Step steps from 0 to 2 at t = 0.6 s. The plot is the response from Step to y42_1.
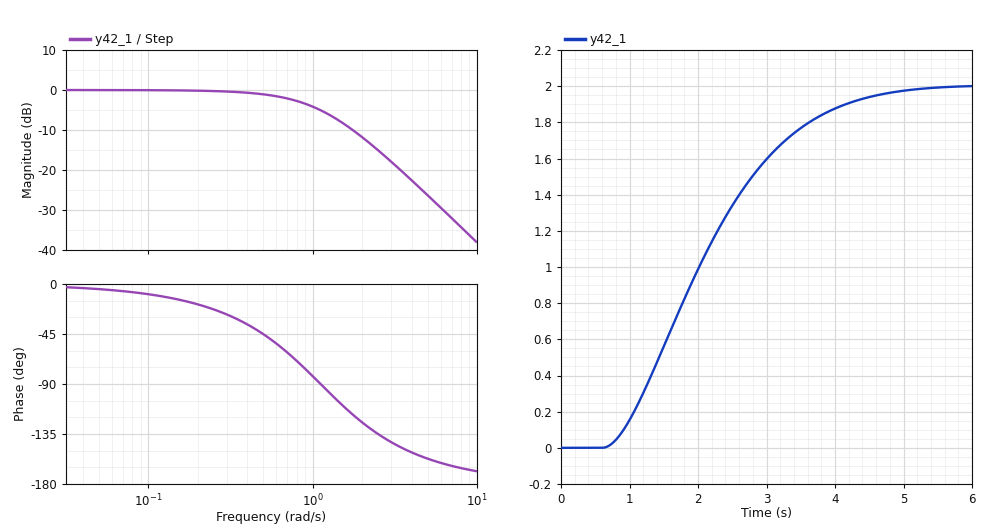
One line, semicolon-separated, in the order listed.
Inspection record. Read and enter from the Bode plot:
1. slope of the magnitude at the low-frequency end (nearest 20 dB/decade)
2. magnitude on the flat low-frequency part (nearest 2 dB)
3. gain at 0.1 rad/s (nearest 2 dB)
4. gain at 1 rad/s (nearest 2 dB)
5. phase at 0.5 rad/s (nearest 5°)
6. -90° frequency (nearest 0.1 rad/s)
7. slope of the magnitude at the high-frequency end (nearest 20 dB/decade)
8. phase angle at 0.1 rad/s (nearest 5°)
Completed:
0 dB/decade; 0 dB; 0 dB; -4 dB; -45°; 1.1 rad/s; -40 dB/decade; -10°
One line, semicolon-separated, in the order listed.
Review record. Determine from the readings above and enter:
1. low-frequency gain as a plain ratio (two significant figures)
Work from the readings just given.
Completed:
1.0
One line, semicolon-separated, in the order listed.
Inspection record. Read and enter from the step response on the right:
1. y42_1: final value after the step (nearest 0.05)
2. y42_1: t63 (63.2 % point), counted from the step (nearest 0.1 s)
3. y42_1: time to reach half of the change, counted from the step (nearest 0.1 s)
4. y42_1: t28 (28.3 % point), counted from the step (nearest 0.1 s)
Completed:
2.00; 1.8 s; 1.4 s; 0.9 s
